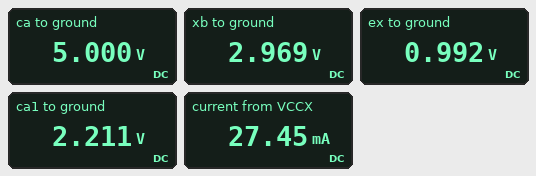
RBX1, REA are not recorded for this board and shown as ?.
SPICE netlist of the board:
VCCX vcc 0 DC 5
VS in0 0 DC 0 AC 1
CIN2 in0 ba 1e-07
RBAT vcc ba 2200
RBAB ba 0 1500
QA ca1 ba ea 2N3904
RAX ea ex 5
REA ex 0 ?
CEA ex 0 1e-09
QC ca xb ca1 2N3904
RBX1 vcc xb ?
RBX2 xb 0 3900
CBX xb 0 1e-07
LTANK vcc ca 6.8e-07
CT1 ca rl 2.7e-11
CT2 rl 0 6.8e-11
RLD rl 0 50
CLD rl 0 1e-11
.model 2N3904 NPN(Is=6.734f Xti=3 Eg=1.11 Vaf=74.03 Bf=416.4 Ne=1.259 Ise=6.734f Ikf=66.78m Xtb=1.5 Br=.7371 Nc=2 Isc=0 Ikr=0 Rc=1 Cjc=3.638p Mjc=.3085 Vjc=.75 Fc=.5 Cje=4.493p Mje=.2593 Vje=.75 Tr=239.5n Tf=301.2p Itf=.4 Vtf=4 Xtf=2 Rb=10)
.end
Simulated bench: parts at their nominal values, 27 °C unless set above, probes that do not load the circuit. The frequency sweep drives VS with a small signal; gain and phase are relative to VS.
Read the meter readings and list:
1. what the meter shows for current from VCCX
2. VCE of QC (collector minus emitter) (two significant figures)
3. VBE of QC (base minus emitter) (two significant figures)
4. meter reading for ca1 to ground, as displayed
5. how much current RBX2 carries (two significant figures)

27.45 mA
2.8 V
760 mV
2.211 V
760 µA
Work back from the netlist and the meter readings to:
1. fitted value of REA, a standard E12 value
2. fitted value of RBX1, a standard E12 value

39 Ω
2.2 kΩ
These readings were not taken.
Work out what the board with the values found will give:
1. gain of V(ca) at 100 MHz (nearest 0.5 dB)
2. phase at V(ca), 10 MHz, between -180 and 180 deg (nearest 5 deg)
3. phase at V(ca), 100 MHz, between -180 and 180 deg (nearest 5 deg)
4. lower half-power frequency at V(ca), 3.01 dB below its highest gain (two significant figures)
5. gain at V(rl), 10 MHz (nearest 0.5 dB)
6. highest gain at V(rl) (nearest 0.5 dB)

21.0 dB
-45 deg
70 deg
36 MHz
-14.0 dB
30.0 dB
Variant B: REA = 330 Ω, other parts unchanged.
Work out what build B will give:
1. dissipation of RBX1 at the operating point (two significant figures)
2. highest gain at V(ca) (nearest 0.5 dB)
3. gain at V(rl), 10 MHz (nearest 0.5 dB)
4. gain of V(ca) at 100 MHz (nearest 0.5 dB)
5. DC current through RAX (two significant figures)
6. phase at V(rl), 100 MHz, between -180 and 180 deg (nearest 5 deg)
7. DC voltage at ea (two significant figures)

1.5 mW
39.5 dB
-15.0 dB
16.0 dB
3.9 mA
90 deg
1.3 V
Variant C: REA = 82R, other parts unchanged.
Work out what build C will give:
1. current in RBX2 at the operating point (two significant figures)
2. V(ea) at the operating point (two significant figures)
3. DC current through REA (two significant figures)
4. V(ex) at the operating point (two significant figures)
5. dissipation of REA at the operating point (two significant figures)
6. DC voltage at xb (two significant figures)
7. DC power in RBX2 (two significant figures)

790 µA
1.2 V
14 mA
1.1 V
16 mW
3.1 V
2.4 mW
